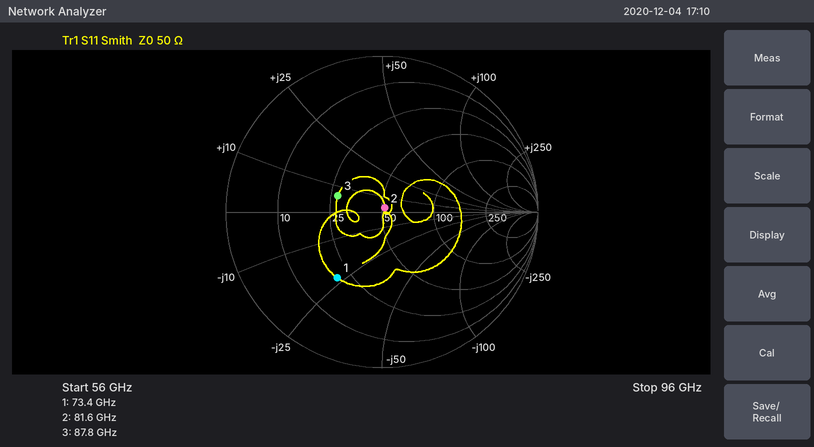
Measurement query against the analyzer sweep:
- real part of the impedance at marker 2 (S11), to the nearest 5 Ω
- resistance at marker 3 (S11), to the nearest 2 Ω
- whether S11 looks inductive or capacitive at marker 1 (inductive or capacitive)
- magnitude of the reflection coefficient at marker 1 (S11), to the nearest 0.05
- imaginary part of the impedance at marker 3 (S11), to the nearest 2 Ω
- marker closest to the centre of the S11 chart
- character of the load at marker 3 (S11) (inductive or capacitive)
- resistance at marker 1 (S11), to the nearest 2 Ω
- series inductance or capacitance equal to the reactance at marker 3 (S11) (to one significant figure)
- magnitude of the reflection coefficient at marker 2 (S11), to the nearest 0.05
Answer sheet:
50 Ω
28 Ω
capacitive
0.50
+6 Ω
marker 2
inductive
20 Ω
10 pH
0.05
